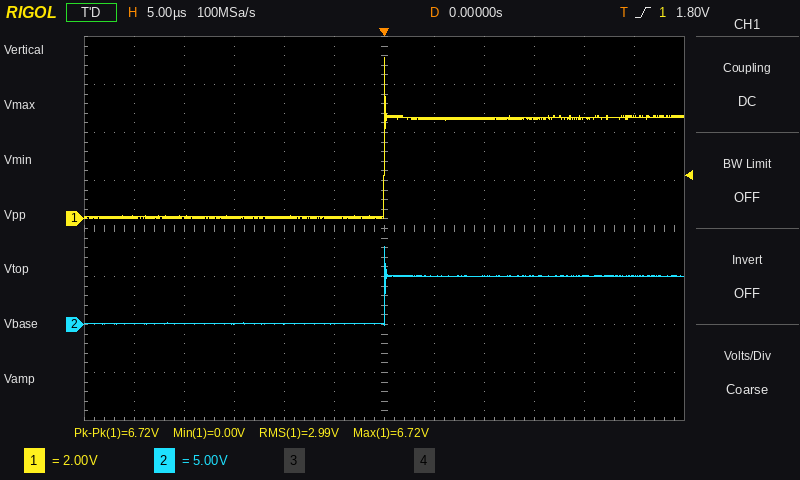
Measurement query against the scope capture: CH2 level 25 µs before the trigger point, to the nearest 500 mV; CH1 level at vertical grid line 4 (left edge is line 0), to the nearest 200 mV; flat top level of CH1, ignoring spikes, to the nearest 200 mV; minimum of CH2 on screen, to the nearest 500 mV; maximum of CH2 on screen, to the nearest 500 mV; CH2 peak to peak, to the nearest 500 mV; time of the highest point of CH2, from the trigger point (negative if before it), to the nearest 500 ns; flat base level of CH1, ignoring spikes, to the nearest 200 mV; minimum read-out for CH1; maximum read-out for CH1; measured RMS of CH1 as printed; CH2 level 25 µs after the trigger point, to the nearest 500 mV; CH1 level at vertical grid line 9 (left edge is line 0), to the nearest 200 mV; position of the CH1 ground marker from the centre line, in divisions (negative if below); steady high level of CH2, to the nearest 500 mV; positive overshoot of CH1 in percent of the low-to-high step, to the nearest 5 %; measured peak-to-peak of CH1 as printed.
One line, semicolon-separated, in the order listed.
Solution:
0.0 V; 0.0 V; 4.2 V; 0.0 V; 8.0 V; 8.0 V; 0.0 µs; 0.0 V; 0.00 V; 6.72 V; 2.99 V; 5.0 V; 4.2 V; +0.2 div; 5.0 V; 60 %; 6.72 V
